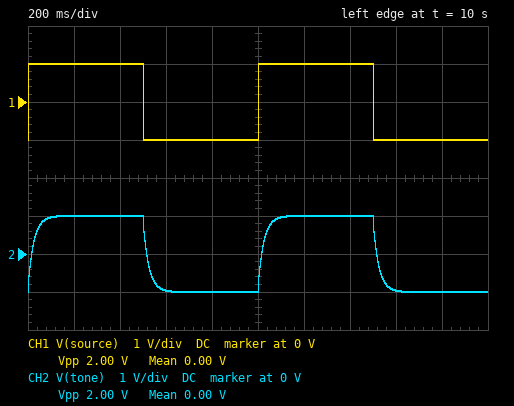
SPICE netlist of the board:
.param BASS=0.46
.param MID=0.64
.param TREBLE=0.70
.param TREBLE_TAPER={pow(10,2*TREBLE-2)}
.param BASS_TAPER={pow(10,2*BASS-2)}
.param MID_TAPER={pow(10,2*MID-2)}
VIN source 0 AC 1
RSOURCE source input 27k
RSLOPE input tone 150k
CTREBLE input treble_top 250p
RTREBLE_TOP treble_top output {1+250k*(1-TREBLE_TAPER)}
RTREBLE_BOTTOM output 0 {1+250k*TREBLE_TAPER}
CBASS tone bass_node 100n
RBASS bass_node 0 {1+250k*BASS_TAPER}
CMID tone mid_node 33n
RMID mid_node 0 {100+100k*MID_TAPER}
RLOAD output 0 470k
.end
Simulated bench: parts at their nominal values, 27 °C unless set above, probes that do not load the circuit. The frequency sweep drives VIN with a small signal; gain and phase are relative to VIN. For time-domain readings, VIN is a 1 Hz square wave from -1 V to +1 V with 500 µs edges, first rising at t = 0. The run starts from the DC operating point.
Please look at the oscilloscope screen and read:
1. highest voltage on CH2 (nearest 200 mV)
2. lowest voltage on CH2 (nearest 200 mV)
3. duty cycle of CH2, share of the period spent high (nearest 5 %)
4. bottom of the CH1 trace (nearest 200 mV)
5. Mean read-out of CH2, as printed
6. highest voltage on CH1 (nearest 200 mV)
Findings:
1.0 V
-1.0 V
50 %
-1.0 V
0.00 V
1.0 V
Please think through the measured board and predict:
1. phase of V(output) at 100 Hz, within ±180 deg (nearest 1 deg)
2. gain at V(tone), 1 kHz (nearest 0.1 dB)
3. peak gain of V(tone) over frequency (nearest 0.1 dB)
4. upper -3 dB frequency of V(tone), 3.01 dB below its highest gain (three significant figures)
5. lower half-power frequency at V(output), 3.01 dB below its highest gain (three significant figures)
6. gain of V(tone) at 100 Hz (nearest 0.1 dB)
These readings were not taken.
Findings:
87 deg
-25.4 dB
0 dB
6.33 Hz
2.40 kHz
-20.5 dB
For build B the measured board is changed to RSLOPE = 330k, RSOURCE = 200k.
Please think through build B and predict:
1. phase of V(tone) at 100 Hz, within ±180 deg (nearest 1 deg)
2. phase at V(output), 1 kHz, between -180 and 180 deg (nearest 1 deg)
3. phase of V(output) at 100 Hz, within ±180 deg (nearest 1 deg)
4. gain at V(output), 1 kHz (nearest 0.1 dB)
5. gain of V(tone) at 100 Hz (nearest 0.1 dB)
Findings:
-47 deg
60 deg
86 deg
-26.5 dB
-29.6 dB
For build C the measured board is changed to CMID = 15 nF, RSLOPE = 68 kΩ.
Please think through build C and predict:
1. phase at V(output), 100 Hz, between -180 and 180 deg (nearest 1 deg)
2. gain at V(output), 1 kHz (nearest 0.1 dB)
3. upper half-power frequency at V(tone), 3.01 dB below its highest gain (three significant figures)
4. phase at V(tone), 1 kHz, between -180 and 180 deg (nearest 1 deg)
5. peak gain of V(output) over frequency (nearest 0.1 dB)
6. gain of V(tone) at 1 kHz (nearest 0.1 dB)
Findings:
85 deg
-24.5 dB
12.8 Hz
-16 deg
-16.1 dB
-19.8 dB
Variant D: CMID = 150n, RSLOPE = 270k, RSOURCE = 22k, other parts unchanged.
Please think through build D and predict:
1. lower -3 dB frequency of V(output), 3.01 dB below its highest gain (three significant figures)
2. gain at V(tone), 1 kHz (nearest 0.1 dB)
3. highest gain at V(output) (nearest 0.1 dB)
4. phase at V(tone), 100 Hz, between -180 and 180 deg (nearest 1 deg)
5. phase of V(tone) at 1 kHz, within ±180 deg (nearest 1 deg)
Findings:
2.42 kHz
-29.7 dB
-14.2 dB
-32 deg
-5 deg
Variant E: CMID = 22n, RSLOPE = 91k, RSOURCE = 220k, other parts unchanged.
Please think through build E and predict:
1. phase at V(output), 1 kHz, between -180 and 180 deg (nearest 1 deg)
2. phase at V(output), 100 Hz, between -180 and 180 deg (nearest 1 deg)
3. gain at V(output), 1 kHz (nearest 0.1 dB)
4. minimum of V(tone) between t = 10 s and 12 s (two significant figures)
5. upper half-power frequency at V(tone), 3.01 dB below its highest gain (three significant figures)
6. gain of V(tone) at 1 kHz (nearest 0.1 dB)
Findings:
63 deg
82 deg
-32.2 dB
-1.0 V
4.01 Hz
-30.1 dB
